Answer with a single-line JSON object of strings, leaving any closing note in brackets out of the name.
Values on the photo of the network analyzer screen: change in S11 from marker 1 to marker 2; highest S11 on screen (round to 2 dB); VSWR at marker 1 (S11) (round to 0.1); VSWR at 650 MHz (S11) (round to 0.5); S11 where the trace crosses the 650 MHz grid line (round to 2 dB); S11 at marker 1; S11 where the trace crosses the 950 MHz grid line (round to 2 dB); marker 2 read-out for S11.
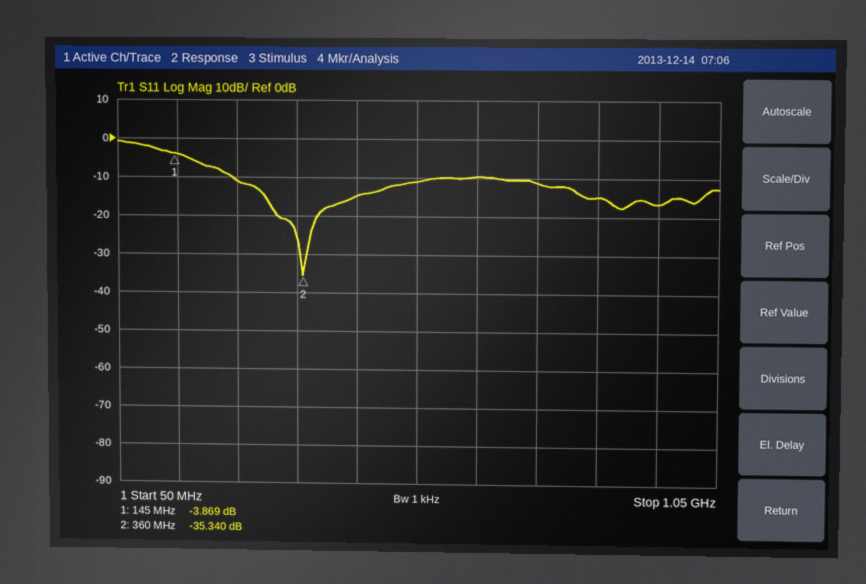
{"change in S11 from marker 1 to marker 2": "-31.471 dB", "highest S11 on screen": "0 dB", "VSWR at marker 1 (S11)": "4.6", "VSWR at 650 MHz (S11)": "2.0", "S11 where the trace crosses the 650 MHz grid line": "-10 dB", "S11 at marker 1": "-3.869 dB", "S11 where the trace crosses the 950 MHz grid line": "-16 dB", "marker 2 read-out for S11": "-35.340 dB"}
